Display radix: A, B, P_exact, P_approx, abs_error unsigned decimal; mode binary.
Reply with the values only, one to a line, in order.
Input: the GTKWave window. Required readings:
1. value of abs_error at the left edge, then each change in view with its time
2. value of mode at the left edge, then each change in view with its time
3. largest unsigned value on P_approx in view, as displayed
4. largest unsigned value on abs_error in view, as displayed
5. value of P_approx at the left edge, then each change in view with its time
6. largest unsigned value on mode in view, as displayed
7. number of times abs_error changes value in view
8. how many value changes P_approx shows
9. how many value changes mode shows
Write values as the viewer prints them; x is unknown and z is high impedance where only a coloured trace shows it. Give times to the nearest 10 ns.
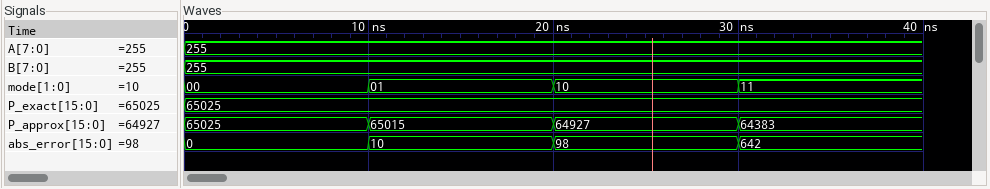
0, 10 at 10 ns, 98 at 20 ns, 642 at 30 ns
00, 01 at 10 ns, 10 at 20 ns, 11 at 30 ns
65025
642
65025, 65015 at 10 ns, 64927 at 20 ns, 64383 at 30 ns
11
3
3
3
